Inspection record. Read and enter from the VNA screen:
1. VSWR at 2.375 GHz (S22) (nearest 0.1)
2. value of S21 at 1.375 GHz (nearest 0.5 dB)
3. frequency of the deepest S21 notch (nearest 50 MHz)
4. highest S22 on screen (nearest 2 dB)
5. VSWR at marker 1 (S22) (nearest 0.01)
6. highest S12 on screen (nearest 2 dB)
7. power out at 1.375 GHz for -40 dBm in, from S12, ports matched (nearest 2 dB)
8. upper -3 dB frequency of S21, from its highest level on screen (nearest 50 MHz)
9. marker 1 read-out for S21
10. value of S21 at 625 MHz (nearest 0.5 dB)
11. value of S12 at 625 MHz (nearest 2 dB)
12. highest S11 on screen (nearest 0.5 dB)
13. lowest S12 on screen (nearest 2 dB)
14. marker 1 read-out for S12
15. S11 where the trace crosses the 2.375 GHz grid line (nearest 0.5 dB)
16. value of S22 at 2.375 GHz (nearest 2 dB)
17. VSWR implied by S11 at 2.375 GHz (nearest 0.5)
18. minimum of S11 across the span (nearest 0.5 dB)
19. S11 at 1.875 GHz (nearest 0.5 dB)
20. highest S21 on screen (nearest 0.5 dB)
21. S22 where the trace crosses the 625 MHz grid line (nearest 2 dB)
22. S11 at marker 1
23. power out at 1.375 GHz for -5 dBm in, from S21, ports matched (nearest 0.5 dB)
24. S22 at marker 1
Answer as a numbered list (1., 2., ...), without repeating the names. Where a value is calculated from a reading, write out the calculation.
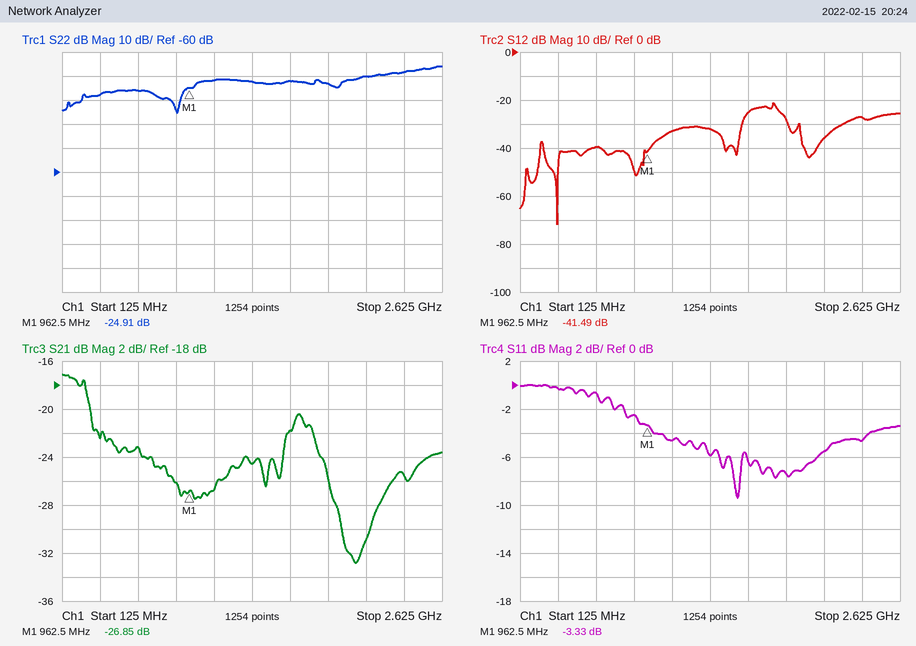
1. |Γ| = 10^(-18/20) = 0.1259; VSWR = (1 + 0.1259)/(1 − 0.1259) ≈ 1.3
2. -24.5 dB
3. 2.05 GHz
4. -16 dB
5. (1 + 0.0568)/(1 − 0.0568) ≈ 1.12
6. -22 dB
7. -40 dBm + (-32 dB) = -72 dBm
8. 300 MHz
9. -26.85 dB
10. -23.0 dB
11. -40 dB
12. 0.0 dB
13. -72 dB
14. -41.49 dB
15. -4.5 dB
16. -18 dB
17. |Γ| = 10^(-4.5/20) = 0.5957; VSWR = (1 + 0.5957)/(1 − 0.5957) ≈ 4.0
18. -9.5 dB
19. -7.5 dB
20. -17.0 dB
21. -26 dB
22. -3.33 dB
23. -5 dBm + (-24.5 dB) = -29.5 dBm
24. -24.91 dB
